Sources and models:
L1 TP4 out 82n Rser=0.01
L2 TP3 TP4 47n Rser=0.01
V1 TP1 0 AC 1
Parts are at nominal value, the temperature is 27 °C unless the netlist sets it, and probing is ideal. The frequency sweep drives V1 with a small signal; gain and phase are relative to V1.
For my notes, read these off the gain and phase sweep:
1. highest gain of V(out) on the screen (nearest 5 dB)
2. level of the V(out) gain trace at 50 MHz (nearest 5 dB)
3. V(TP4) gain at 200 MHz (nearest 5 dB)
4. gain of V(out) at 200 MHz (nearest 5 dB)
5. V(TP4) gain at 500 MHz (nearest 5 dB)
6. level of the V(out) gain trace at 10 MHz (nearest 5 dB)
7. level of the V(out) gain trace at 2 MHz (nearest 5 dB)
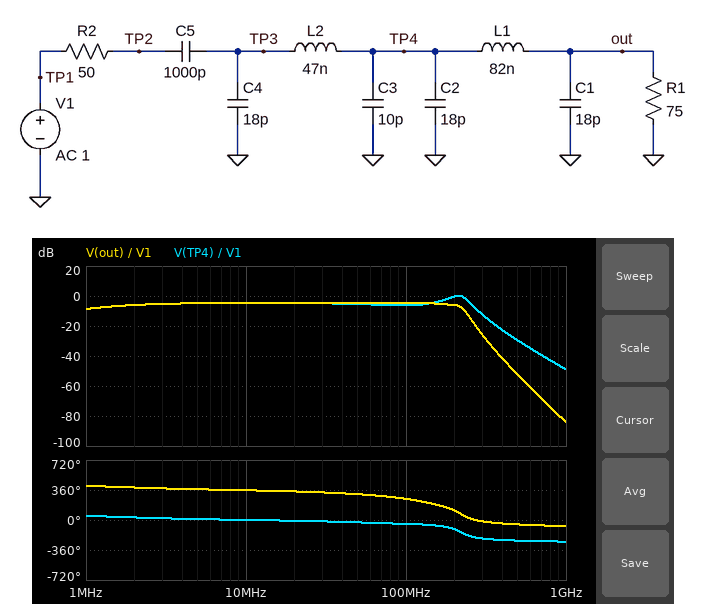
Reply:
-5 dB
-5 dB
0 dB
-5 dB
-30 dB
-5 dB
-5 dB
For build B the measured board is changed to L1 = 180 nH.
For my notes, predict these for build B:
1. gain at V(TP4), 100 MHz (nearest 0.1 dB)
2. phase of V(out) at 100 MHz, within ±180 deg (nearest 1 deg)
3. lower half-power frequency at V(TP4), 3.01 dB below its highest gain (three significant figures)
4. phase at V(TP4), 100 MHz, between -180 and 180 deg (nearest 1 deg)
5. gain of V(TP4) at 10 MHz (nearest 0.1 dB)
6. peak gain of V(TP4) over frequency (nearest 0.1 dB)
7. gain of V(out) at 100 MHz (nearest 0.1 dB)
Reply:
-2.9 dB
-145 deg
97.1 MHz
-45 deg
-4.6 dB
0 dB
-6.6 dB
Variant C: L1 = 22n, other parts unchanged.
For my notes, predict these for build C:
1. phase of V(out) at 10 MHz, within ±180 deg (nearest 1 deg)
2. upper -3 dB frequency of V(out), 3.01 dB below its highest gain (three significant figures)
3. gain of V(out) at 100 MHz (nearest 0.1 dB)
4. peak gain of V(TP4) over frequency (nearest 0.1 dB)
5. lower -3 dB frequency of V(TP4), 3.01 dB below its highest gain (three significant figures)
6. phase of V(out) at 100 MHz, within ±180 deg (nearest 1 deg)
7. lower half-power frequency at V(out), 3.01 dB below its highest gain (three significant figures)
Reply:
-2 deg
217 MHz
-5.4 dB
-4.7 dB
1.22 MHz
-79 deg
1.23 MHz
